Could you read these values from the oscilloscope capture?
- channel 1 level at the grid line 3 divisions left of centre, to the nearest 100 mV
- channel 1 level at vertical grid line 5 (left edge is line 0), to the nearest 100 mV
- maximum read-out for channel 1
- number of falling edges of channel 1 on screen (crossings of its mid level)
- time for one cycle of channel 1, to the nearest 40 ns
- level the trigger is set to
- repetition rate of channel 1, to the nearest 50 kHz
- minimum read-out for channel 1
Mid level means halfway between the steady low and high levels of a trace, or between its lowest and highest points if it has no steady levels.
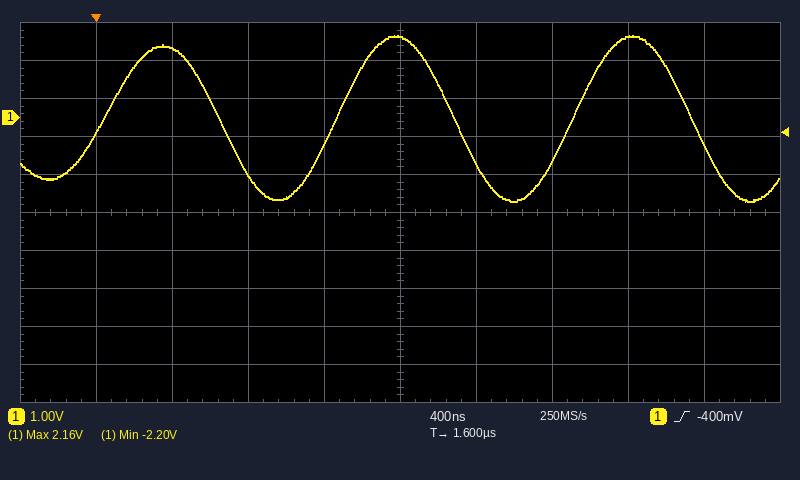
1.8 V
2.1 V
2.16 V
3
1.24 µs
-400 mV
800 kHz
-2.20 V
